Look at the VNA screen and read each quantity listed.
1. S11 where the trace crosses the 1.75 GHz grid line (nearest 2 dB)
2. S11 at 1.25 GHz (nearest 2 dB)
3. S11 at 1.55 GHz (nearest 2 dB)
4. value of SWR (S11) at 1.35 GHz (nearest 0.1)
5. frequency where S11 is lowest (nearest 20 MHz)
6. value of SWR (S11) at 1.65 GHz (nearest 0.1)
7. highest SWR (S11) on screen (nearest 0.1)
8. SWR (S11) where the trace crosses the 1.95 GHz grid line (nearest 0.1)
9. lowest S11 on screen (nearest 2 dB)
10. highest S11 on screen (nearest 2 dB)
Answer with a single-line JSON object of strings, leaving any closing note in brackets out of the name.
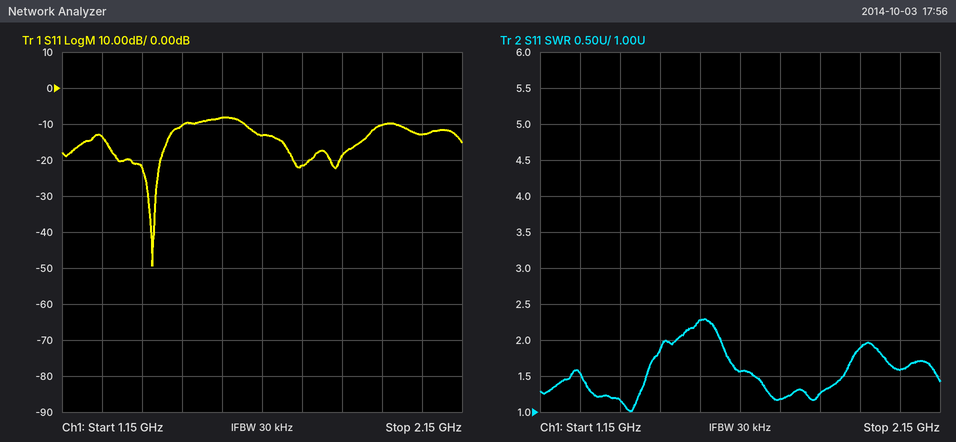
{"S11 where the trace crosses the 1.75 GHz grid line": "-22 dB", "S11 at 1.25 GHz": "-14 dB", "S11 at 1.55 GHz": "-8 dB", "value of SWR (S11) at 1.35 GHz": "1.2", "frequency where S11 is lowest": "1.38 GHz", "value of SWR (S11) at 1.65 GHz": "1.6", "highest SWR (S11) on screen": "2.3", "SWR (S11) where the trace crosses the 1.95 GHz grid line": "1.9", "lowest S11 on screen": "-50 dB", "highest S11 on screen": "-8 dB"}
